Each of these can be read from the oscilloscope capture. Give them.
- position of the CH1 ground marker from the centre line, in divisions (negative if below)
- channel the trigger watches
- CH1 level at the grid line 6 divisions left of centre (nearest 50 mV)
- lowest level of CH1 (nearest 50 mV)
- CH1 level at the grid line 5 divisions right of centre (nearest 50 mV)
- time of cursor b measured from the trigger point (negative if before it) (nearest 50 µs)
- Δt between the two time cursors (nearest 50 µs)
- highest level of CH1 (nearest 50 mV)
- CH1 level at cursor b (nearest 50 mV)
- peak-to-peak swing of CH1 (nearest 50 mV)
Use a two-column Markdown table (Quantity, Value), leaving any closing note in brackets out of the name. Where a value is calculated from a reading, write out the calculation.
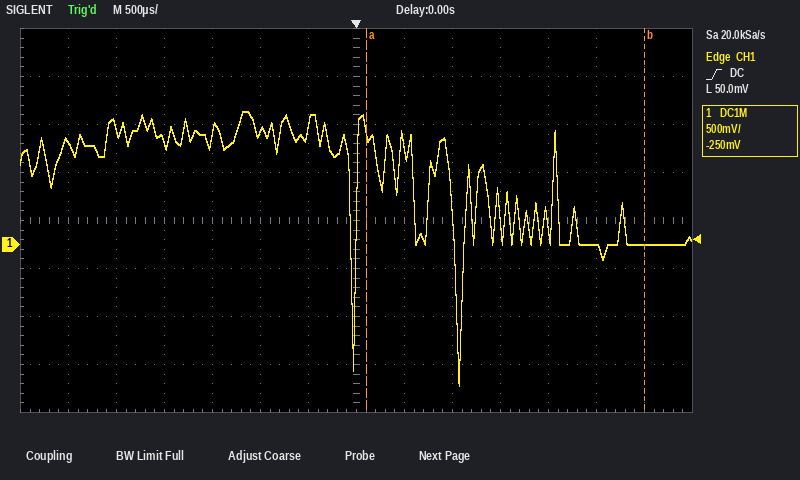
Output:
| Quantity | Value |
|---|---|
| position of the CH1 ground marker from the centre line, in divisions | -0.5 div |
| channel the trigger watches | CH1 |
| CH1 level at the grid line 6 divisions left of centre | 1.05 V |
| lowest level of CH1 | -1.45 V |
| CH1 level at the grid line 5 divisions right of centre | 0 mV |
| time of cursor b measured from the trigger point (negative if before it) | +3.00 ms |
| Δt between the two time cursors | 2.90 ms |
| highest level of CH1 | 1.40 V |
| CH1 level at cursor b | 0 mV |
| peak-to-peak swing of CH1 | 1.40 V − (-1.45 V) = 2.85 V |
